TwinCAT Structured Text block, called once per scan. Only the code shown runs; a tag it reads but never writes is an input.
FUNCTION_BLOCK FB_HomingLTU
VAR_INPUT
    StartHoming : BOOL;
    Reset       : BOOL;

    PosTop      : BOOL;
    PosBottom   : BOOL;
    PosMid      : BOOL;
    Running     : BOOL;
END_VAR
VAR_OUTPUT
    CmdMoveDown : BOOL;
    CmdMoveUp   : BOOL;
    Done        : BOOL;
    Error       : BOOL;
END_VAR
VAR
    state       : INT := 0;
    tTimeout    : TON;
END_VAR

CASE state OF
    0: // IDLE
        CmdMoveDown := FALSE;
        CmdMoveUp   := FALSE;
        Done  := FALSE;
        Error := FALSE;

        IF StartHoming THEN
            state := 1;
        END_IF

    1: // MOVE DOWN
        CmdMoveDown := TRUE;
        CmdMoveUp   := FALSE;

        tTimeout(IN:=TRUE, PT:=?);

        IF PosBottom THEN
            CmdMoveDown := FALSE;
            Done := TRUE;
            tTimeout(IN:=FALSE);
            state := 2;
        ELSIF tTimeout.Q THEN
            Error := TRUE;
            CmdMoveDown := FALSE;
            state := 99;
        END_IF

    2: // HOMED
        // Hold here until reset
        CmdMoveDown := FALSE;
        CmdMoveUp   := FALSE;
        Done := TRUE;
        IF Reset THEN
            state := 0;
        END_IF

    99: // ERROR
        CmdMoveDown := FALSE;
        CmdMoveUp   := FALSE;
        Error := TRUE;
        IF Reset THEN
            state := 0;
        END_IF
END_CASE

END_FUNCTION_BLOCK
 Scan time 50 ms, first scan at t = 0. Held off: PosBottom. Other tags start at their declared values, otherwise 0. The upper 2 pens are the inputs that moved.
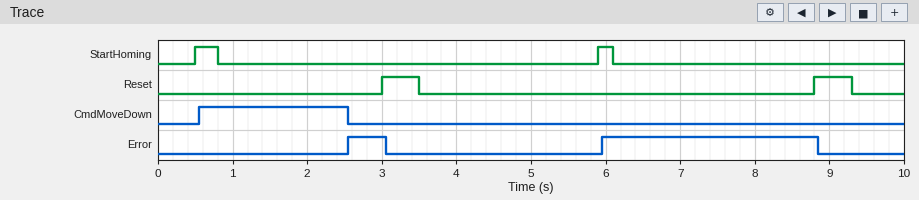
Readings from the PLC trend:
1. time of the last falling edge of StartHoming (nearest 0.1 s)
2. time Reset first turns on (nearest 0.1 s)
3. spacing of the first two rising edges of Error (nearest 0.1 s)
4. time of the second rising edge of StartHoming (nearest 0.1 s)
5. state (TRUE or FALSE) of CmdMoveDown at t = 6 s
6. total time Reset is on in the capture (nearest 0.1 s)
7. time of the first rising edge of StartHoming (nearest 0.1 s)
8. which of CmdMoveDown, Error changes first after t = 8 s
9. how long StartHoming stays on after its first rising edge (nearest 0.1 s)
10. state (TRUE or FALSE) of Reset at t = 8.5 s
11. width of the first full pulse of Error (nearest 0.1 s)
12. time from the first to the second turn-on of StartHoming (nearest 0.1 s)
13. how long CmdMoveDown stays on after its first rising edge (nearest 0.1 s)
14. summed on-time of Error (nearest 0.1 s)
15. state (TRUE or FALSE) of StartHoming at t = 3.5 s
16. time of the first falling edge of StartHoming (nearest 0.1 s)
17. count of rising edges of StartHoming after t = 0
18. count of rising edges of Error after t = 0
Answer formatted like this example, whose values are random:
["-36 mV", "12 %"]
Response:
["6.1 s", "3.0 s", "3.4 s", "5.9 s", "FALSE", "1.0 s", "0.5 s", "Error", "0.3 s", "FALSE", "0.5 s", "5.4 s", "2.0 s", "3.4 s", "FALSE", "0.8 s", "2", "2"]
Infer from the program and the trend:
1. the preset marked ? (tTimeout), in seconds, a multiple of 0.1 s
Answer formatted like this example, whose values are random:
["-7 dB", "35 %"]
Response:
["2.0 s"]
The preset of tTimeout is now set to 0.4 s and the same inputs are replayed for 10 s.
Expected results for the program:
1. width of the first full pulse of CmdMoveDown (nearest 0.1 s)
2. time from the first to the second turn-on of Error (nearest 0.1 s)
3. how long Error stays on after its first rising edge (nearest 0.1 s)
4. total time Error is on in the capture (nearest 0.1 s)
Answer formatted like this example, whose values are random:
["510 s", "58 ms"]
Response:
["0.4 s", "5.0 s", "2.1 s", "5.0 s"]
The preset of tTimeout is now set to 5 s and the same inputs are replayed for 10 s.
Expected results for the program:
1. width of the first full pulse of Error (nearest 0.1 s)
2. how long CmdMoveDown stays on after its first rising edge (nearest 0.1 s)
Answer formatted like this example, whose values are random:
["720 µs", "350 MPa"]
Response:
["3.3 s", "5.0 s"]
